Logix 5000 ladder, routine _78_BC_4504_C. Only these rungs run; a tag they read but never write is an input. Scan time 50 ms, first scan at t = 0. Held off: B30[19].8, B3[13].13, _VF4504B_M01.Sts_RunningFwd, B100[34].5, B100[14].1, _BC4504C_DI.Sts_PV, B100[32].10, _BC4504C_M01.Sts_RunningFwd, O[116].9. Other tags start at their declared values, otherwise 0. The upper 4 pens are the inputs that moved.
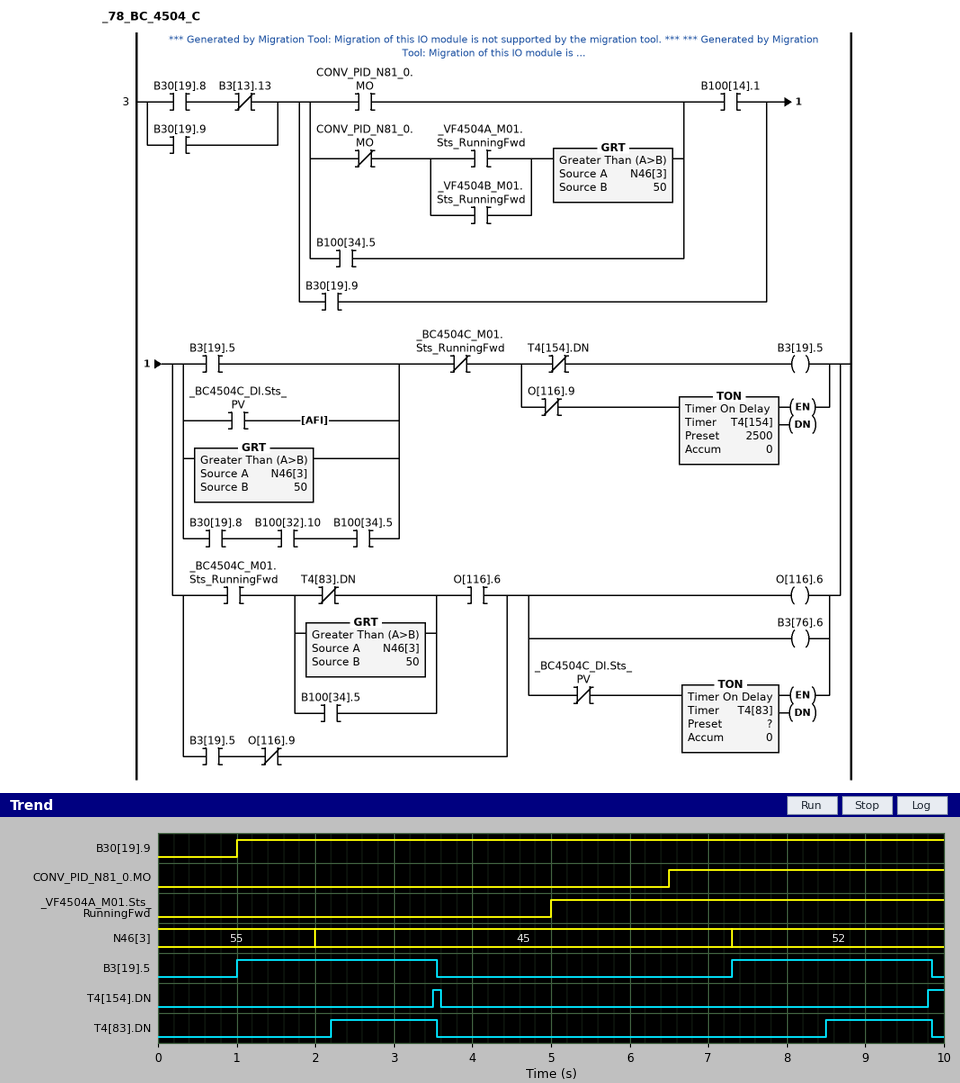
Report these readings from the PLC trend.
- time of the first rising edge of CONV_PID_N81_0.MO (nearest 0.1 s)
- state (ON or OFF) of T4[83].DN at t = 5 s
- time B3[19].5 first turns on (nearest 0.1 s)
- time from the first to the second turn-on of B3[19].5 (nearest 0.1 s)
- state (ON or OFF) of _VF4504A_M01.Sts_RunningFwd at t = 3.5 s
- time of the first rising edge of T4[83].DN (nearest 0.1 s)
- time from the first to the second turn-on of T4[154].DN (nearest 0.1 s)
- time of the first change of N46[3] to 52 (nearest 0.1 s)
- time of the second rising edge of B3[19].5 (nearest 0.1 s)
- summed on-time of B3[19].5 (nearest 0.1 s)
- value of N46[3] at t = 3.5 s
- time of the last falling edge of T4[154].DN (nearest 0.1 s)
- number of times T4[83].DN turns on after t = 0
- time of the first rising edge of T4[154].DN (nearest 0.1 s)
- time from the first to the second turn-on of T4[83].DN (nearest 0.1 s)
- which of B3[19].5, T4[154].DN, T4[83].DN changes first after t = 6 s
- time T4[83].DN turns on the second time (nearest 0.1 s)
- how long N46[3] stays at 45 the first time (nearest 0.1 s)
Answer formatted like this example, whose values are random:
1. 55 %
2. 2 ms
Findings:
1. 6.5 s
2. OFF
3. 1.0 s
4. 6.3 s
5. OFF
6. 2.2 s
7. 6.3 s
8. 7.3 s
9. 7.3 s
10. 5.1 s
11. 45
12. 3.6 s
13. 2
14. 3.5 s
15. 6.3 s
16. B3[19].5
17. 8.5 s
18. 5.3 s
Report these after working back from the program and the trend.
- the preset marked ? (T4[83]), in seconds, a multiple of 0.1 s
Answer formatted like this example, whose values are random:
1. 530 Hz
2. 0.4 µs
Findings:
1. 1.2 s
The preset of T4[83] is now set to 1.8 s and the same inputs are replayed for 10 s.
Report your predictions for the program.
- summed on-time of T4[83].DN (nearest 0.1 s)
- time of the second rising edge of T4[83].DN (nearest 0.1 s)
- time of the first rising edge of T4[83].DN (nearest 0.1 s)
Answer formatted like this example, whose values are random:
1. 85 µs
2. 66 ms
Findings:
1. 1.5 s
2. 9.1 s
3. 2.8 s
